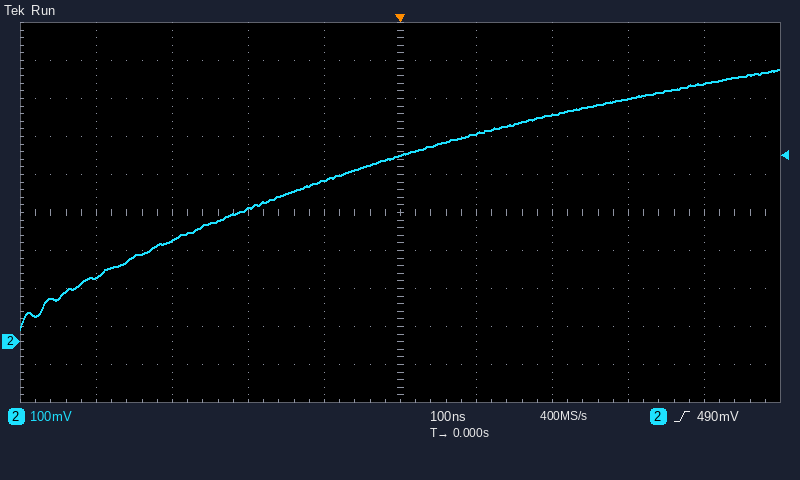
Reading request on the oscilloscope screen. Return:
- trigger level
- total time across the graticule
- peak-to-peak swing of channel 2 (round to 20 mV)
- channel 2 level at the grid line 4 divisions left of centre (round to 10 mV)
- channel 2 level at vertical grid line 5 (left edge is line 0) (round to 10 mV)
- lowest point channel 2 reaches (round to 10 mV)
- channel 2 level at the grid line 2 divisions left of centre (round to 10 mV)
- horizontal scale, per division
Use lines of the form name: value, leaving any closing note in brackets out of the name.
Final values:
trigger level: 490 mV
total time across the graticule: 1 µs
peak-to-peak swing of channel 2: 680 mV
channel 2 level at the grid line 4 divisions left of centre: 170 mV
channel 2 level at vertical grid line 5 (left edge is line 0): 490 mV
lowest point channel 2 reaches: 30 mV
channel 2 level at the grid line 2 divisions left of centre: 350 mV
horizontal scale, per division: 100 ns
